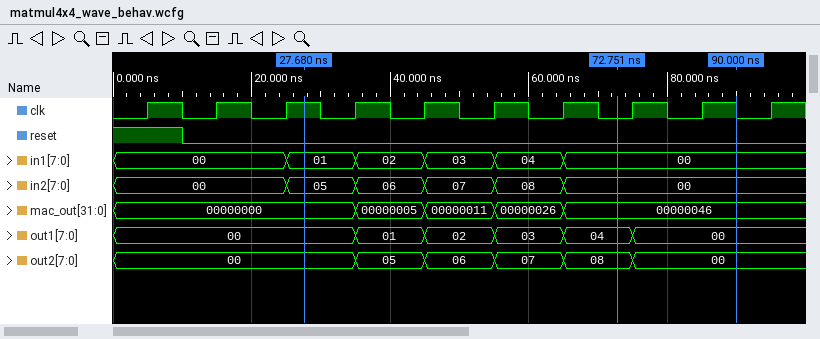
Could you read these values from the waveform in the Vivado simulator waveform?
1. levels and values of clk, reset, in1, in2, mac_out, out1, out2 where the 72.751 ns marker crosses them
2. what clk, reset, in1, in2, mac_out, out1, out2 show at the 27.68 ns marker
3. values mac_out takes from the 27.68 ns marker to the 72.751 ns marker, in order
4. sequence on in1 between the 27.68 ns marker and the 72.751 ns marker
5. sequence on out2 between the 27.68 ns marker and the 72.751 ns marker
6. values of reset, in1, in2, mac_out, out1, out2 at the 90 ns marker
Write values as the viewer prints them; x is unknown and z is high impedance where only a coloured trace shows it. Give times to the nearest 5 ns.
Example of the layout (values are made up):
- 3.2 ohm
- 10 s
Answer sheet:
- clk=0, reset=0, in1=00, in2=00, mac_out=00000046, out1=04, out2=08
- clk=1, reset=0, in1=01, in2=05, mac_out=00000000, out1=00, out2=00
- 00000000, 00000005, 00000011, 00000026, 00000046
- 01, 02, 03, 04, 00
- 00, 05, 06, 07, 08
- reset=0, in1=00, in2=00, mac_out=00000046, out1=00, out2=00
